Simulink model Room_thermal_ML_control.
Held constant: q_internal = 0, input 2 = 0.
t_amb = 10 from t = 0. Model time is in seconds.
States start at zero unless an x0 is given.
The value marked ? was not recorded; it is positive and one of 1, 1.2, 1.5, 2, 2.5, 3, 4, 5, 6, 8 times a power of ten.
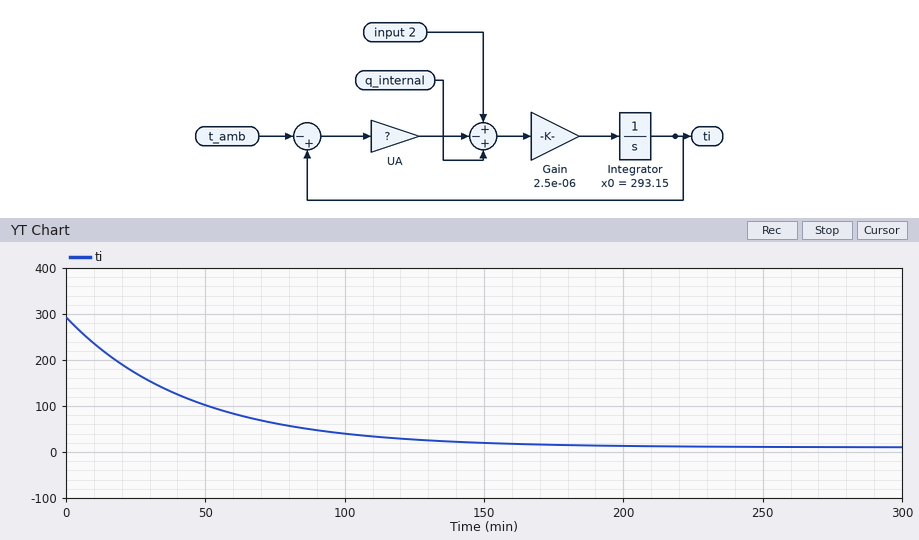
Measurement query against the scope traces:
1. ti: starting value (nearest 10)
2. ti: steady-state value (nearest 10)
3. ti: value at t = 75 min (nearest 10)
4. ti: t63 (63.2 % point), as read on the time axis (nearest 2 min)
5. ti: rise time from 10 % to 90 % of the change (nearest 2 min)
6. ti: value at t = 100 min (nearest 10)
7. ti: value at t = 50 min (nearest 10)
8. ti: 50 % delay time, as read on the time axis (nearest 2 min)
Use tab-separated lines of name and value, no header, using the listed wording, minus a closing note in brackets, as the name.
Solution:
ti: starting value	290
ti: steady-state value	10
ti: value at t = 75 min	60
ti: t63 (63.2 % point), as read on the time axis	44 min
ti: rise time from 10 % to 90 % of the change	98 min
ti: value at t = 100 min	40
ti: value at t = 50 min	100
ti: 50 % delay time, as read on the time axis	30 min
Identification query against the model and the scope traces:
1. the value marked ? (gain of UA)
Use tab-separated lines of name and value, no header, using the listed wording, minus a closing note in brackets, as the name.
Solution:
the value marked ?	150
